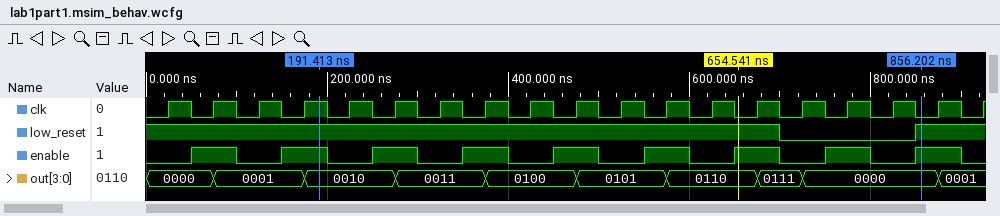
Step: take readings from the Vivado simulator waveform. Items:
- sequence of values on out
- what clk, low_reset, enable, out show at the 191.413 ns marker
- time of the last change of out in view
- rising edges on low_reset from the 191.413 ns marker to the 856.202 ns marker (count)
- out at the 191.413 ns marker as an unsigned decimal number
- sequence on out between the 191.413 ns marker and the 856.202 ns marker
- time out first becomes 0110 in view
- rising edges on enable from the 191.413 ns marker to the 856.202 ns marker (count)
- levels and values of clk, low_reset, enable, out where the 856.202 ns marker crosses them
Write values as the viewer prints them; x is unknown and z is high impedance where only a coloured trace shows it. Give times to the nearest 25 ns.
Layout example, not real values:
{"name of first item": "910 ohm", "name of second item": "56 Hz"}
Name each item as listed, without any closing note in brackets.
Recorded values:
{"sequence of values on out": "0000, 0001, 0010, 0011, 0100, 0101, 0110, 0111, 0000, 0001", "what clk, low_reset, enable, out show at the 191.413 ns marker": "clk=1, low_reset=1, enable=1, out=0010", "time of the last change of out in view": "875 ns", "rising edges on low_reset from the 191.413 ns marker to the 856.202 ns marker": "1", "out at the 191.413 ns marker as an unsigned decimal number": "2", "sequence on out between the 191.413 ns marker and the 856.202 ns marker": "0010, 0011, 0100, 0101, 0110, 0111, 0000", "time out first becomes 0110 in view": "575 ns", "rising edges on enable from the 191.413 ns marker to the 856.202 ns marker": "7", "levels and values of clk, low_reset, enable, out where the 856.202 ns marker crosses them": "clk=0, low_reset=1, enable=1, out=0000"}
